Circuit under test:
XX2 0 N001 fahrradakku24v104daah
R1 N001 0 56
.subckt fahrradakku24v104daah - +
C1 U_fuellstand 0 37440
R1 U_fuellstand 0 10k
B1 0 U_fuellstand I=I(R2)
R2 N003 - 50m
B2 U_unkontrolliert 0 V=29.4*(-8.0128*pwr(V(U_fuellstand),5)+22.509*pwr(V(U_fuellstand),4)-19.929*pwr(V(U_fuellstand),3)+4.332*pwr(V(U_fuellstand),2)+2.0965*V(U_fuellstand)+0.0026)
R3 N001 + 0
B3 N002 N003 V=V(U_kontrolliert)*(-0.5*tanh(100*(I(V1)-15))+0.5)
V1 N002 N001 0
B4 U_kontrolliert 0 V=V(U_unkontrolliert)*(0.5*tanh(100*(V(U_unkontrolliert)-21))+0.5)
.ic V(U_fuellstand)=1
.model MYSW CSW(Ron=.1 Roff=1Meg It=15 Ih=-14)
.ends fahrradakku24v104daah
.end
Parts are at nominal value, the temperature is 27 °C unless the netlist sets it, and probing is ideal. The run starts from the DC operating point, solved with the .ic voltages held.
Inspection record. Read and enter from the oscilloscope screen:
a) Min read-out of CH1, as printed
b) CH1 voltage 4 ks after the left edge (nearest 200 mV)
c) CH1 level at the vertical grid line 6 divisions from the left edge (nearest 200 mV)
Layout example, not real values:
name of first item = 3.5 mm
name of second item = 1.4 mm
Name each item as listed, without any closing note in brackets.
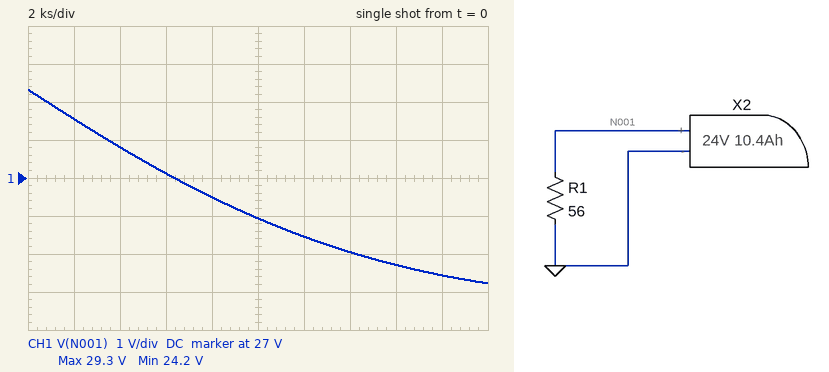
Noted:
Min read-out of CH1, as printed = 24.2 V
CH1 voltage 4 ks after the left edge = 27.8 V
CH1 level at the vertical grid line 6 divisions from the left edge = 25.4 V
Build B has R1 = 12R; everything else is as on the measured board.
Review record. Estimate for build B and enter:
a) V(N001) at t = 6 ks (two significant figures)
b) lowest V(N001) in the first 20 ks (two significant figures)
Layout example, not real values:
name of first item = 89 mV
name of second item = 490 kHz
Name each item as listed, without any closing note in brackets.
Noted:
V(N001) at t = 6 ks = 24 V
lowest V(N001) in the first 20 ks = 9.0 mV
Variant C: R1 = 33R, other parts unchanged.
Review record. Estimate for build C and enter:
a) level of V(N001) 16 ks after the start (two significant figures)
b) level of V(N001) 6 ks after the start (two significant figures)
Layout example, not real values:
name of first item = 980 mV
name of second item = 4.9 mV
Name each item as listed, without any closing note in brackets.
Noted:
level of V(N001) 16 ks after the start = 24 V
level of V(N001) 6 ks after the start = 26 V
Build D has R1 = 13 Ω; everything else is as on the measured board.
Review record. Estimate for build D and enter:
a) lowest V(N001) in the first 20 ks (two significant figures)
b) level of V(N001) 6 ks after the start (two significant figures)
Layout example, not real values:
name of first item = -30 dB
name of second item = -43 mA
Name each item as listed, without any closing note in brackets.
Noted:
lowest V(N001) in the first 20 ks = 11 mV
level of V(N001) 6 ks after the start = 24 V
